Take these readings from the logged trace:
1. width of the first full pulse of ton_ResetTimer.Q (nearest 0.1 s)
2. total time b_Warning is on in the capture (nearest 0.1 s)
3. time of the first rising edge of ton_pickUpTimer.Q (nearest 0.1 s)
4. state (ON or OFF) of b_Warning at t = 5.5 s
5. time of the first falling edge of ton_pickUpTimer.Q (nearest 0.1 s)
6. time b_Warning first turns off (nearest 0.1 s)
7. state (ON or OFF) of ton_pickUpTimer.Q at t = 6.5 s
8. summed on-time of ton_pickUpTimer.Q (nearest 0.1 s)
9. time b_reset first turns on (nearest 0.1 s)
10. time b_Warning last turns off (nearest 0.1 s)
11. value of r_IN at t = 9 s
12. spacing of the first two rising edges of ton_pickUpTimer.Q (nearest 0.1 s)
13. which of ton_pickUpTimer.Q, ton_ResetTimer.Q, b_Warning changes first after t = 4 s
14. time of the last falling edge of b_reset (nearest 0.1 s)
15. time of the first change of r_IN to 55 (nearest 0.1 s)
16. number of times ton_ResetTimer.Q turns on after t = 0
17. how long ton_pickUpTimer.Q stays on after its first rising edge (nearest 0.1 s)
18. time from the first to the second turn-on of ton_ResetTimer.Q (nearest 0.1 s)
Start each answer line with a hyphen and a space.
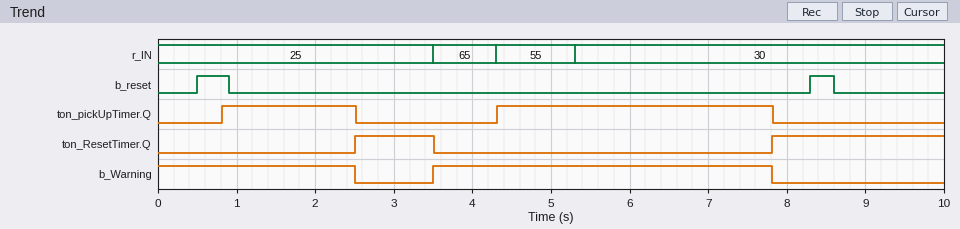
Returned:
- 1.0 s
- 6.8 s
- 0.8 s
- ON
- 2.5 s
- 2.5 s
- ON
- 5.2 s
- 0.5 s
- 7.8 s
- 30
- 3.5 s
- ton_pickUpTimer.Q
- 8.6 s
- 4.3 s
- 2
- 1.7 s
- 5.3 s
